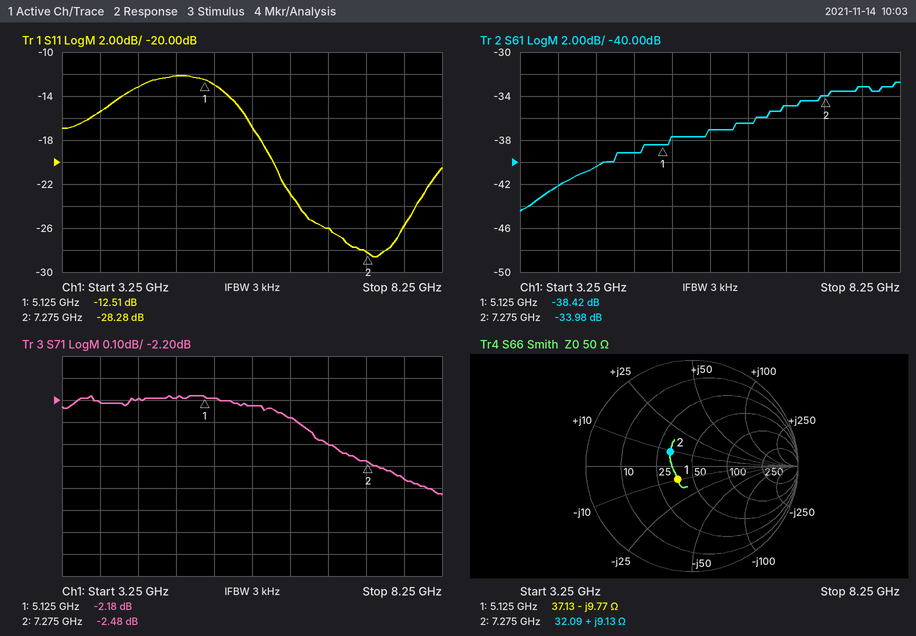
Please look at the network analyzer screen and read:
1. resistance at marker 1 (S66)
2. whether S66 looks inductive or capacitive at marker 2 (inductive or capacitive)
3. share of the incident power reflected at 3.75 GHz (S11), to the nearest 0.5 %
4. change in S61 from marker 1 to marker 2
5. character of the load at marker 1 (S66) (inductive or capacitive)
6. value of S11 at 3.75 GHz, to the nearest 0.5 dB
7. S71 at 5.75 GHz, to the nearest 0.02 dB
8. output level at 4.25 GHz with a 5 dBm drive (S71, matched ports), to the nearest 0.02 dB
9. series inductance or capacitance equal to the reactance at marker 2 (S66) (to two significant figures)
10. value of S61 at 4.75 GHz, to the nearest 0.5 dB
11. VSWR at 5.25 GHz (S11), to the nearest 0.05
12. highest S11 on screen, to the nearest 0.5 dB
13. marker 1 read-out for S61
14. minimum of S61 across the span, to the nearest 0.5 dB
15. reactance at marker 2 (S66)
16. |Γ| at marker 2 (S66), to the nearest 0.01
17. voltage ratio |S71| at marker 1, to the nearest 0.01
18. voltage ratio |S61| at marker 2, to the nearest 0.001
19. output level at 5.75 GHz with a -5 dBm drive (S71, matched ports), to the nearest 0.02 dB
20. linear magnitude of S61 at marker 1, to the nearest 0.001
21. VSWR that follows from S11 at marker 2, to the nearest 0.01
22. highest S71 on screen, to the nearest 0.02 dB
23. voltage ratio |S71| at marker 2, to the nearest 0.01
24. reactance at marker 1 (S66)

37.13 Ω
inductive
3.0 %
4.44 dB
capacitive
-15.5 dB
-2.22 dB
2.80 dBm
200 pH
-39.0 dB
1.60
-12.0 dB
-38.42 dB
-44.5 dB
+9.13 Ω
0.24
0.78
0.020
-7.22 dBm
0.012
1.08
-2.18 dB
0.75
-9.77 Ω
